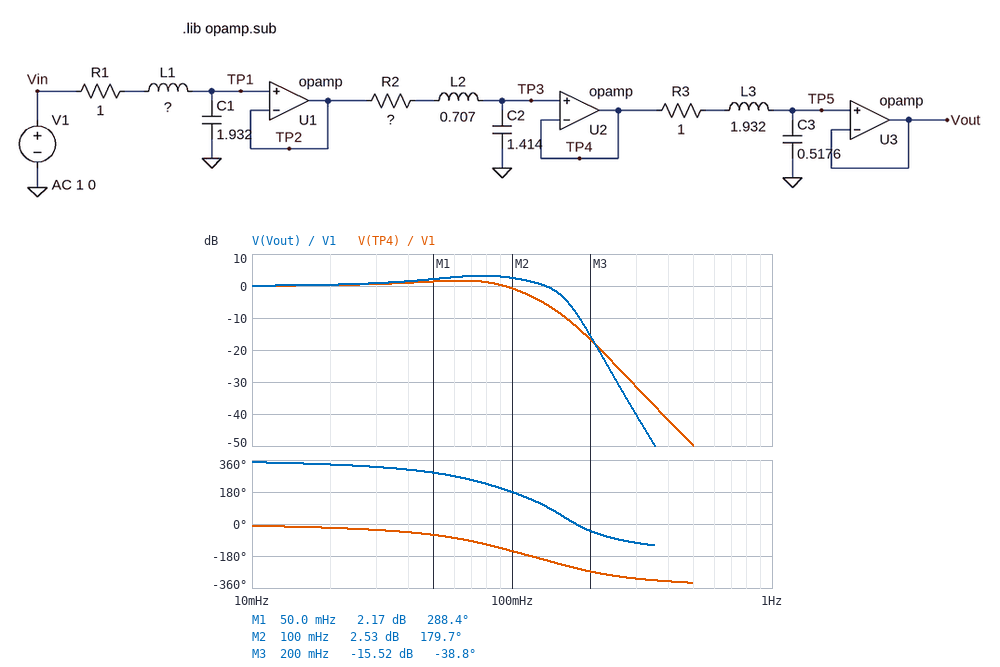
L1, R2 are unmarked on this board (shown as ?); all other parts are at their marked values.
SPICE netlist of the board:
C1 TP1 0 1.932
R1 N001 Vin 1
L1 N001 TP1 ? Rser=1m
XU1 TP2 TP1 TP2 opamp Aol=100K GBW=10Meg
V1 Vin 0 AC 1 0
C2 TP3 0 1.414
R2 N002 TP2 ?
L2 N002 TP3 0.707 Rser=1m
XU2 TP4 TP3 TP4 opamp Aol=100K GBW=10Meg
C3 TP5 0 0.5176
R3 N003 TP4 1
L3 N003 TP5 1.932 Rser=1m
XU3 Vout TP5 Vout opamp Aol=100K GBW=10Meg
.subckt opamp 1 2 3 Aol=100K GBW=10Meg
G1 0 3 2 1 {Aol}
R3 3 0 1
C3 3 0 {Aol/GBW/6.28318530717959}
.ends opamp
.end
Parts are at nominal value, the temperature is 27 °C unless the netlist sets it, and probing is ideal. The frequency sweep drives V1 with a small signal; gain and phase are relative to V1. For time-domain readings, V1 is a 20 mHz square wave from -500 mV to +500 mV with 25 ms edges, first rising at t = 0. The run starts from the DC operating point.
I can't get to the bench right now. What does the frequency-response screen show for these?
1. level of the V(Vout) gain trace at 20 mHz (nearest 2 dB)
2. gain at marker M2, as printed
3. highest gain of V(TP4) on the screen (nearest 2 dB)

0 dB
2.53 dB
2 dB
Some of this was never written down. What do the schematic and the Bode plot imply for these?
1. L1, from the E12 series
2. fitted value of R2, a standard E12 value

1.8 H
0.68 Ω
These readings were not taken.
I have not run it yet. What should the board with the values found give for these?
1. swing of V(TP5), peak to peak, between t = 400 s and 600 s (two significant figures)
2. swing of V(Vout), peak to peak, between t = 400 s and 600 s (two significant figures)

1.8 V
1.8 V
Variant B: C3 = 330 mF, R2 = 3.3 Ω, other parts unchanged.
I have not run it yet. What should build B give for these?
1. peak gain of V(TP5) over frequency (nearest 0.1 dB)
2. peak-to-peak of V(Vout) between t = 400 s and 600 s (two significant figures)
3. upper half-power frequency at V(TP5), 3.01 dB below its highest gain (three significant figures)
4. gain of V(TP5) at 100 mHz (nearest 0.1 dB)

0 dB
990 mV
47.0 mHz
-9.4 dB
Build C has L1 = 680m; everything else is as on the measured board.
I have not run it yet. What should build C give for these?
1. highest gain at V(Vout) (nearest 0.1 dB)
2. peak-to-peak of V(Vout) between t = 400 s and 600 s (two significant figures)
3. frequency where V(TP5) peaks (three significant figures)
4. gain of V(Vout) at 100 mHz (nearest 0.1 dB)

2.8 dB
1.6 V
125 mHz
2.3 dB
